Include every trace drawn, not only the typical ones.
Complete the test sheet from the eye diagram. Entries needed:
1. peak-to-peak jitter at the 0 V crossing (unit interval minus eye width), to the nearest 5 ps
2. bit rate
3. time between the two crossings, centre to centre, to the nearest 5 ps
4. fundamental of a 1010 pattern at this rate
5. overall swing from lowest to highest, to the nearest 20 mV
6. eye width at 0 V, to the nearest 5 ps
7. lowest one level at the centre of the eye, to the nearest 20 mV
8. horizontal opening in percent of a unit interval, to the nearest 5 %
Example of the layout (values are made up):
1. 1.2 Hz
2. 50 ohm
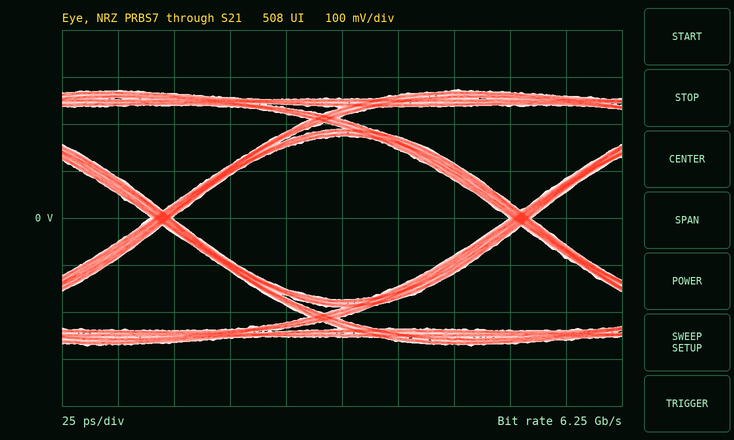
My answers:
1. 10 ps
2. 6.25 Gb/s
3. 160 ps
4. 3.125 GHz
5. 540 mV
6. 150 ps
7. 180 mV
8. 95 %
